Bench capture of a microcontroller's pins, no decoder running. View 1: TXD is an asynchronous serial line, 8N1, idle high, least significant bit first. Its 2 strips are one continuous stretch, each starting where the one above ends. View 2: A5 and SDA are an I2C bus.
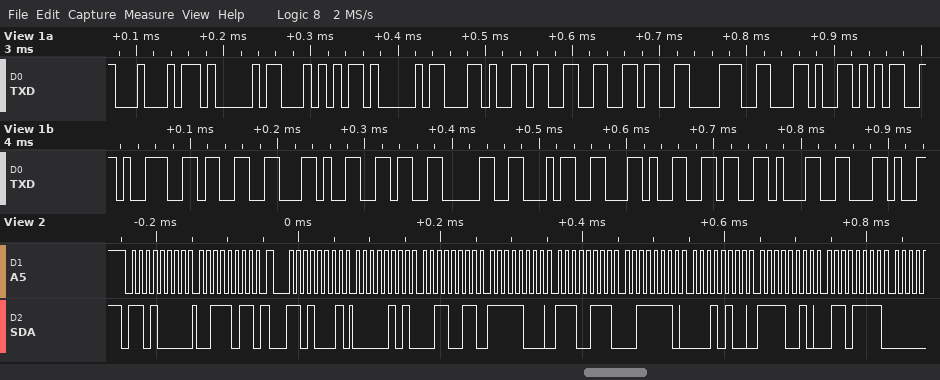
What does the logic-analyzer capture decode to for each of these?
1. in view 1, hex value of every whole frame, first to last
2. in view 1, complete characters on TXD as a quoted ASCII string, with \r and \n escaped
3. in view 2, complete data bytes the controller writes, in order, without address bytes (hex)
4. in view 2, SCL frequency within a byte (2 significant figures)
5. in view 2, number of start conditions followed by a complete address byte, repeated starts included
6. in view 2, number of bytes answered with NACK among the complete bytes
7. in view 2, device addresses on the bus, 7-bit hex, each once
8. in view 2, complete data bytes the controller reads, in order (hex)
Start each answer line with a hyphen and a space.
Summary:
- 0x44 0x41 0x54 0x41 0x2C 0x33 0x36 0x38 0x2C 0x35 0x39 0x33 0x2C 0x36 0x30 0x34 0x2C 0x36 0x31 0x2C
- "DATA,368,593,604,61,"
- 3B
- 100 kHz
- 2
- 0
- 0x68
- 05 33 F8 E7 3E 14 F2 6F
